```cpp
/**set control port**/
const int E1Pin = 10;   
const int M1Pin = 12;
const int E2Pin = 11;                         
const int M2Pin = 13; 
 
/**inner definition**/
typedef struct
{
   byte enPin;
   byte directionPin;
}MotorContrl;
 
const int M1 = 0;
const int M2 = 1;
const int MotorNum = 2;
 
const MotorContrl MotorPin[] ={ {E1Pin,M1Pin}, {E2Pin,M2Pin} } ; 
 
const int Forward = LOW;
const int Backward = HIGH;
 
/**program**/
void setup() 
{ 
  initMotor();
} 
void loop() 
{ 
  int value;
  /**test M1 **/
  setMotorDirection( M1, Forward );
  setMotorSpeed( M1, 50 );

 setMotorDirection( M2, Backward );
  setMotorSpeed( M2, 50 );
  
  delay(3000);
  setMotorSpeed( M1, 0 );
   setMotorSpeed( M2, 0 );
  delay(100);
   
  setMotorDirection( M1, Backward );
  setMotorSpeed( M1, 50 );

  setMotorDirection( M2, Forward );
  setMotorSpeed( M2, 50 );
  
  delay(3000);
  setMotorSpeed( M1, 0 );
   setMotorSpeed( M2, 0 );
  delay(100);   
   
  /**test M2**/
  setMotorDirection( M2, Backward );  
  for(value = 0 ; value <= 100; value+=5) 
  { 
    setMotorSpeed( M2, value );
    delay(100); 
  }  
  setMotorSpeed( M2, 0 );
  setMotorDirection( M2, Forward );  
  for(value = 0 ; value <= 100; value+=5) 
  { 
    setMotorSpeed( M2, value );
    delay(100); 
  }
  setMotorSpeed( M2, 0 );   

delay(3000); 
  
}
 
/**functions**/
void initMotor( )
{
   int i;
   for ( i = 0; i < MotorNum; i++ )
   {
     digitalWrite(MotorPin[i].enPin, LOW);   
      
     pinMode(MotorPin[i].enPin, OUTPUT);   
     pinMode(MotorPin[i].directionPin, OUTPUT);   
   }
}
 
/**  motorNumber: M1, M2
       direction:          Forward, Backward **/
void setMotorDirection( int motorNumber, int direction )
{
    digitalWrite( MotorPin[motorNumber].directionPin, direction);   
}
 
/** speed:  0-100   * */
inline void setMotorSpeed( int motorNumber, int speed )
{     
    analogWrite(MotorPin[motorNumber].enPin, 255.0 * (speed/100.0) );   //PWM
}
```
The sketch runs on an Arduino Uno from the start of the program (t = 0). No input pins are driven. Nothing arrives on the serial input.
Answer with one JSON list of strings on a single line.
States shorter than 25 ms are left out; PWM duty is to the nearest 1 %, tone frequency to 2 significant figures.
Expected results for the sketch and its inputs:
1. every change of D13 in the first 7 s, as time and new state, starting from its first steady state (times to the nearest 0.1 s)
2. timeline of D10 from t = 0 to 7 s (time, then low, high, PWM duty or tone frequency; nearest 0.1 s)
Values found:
["0 s high; 3.1 s low; 6.2 s high", "0 s PWM 50 %; 3 s low; 3.1 s PWM 50 %; 6.1 s low"]
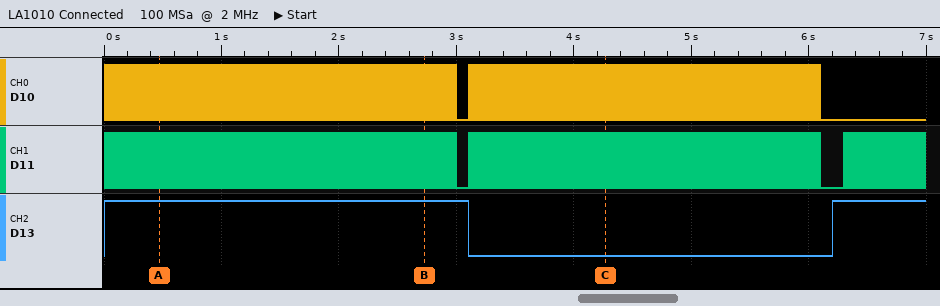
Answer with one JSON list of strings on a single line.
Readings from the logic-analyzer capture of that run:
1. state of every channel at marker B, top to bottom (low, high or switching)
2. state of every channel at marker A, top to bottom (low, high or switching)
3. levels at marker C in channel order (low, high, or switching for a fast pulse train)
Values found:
["D10 switching, D11 switching, D13 high", "D10 switching, D11 switching, D13 high", "D10 switching, D11 switching, D13 low"]
